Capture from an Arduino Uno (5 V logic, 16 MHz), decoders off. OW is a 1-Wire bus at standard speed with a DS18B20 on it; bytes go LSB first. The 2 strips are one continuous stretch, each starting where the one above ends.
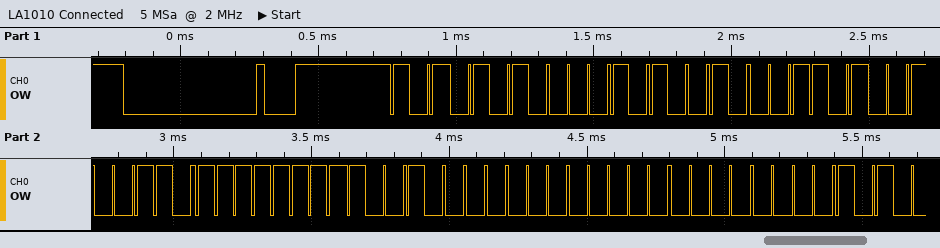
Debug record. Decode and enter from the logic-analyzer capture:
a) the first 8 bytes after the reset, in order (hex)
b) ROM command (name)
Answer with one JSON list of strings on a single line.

["55 28 B1 64 FF 09 00 00", "Match ROM"]
